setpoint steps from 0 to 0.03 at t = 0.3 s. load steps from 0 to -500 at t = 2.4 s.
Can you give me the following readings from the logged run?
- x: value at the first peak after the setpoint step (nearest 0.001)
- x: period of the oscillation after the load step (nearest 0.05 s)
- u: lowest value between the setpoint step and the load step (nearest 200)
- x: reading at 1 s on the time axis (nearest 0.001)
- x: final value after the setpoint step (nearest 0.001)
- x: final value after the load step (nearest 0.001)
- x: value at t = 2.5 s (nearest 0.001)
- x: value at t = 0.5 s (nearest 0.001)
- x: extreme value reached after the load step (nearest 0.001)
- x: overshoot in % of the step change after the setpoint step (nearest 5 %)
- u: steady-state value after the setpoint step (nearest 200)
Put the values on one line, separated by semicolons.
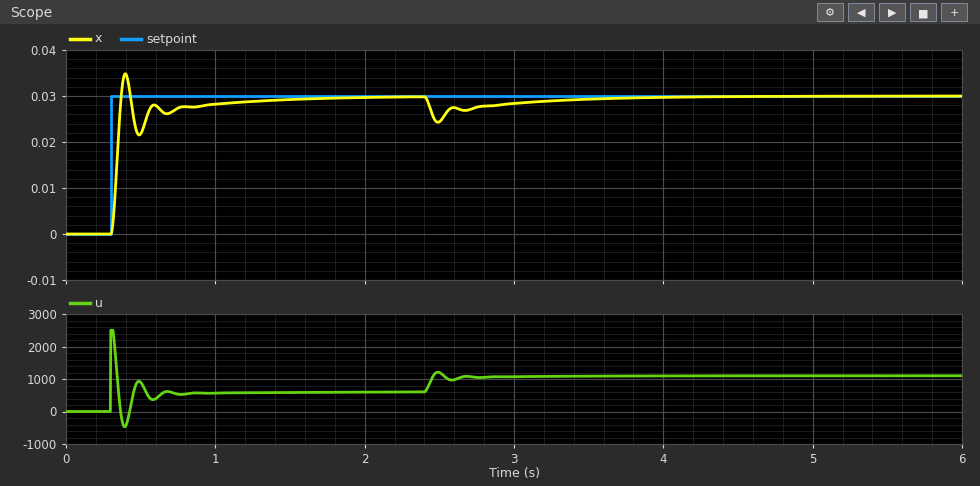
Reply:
0.035; 0.20 s; -400; 0.028; 0.030; 0.030; 0.024; 0.022; 0.024; 15 %; 600
